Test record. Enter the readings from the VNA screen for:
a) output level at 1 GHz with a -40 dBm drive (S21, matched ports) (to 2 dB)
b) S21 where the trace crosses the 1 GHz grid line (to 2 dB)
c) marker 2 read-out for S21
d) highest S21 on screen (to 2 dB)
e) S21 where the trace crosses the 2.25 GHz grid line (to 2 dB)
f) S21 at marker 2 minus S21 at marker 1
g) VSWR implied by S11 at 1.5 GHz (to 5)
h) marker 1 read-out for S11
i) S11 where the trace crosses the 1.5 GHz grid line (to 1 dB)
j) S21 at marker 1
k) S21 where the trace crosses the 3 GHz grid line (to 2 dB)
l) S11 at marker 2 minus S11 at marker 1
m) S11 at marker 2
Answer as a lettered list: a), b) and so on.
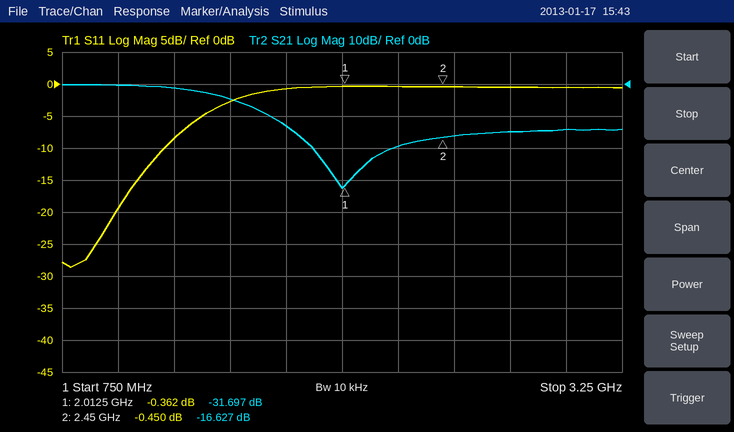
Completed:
a) -40 dBm
b) 0 dB
c) -16.627 dB
d) 0 dB
e) -20 dB
f) 15.070 dB
g) 5
h) -0.362 dB
i) -3 dB
j) -31.697 dB
k) -14 dB
l) -0.088 dB
m) -0.450 dB
